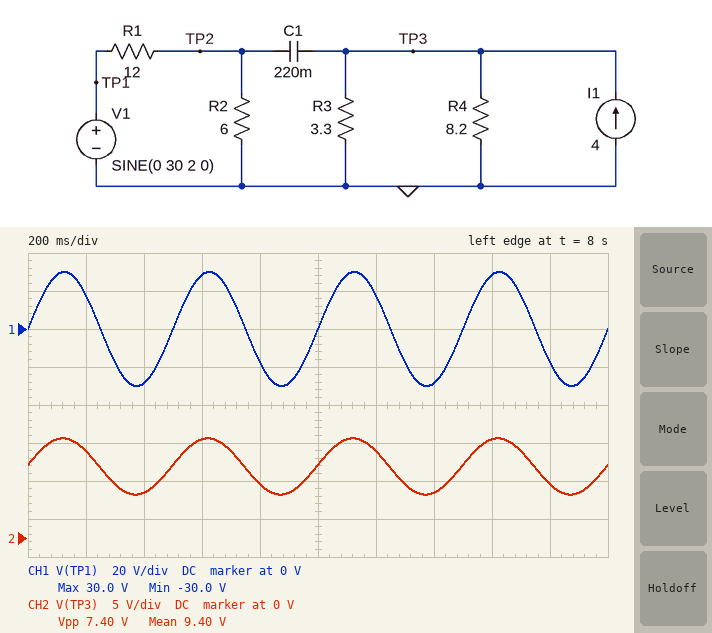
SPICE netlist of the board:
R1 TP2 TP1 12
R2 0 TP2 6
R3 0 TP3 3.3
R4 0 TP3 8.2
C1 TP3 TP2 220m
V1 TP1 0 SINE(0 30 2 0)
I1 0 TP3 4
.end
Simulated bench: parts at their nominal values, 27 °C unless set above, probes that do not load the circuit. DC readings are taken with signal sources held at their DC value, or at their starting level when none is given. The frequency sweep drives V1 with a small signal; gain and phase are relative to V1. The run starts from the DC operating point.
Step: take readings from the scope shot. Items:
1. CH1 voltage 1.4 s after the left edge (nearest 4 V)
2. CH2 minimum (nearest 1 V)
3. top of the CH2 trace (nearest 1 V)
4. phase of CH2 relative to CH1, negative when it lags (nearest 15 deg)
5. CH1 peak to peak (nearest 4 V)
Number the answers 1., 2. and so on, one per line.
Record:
1. -28 V
2. 6 V
3. 13 V
4. 0 deg
5. 60 V
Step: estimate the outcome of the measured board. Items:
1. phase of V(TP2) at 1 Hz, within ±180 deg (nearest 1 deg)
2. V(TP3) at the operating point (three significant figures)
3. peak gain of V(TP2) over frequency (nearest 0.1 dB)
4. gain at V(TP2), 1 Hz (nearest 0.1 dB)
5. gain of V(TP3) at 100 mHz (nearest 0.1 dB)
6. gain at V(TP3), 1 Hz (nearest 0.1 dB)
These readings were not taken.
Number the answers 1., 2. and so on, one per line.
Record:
1. -11 deg
2. 9.41 V
3. -9.5 dB
4. -17.8 dB
5. -21.8 dB
6. -18.2 dB
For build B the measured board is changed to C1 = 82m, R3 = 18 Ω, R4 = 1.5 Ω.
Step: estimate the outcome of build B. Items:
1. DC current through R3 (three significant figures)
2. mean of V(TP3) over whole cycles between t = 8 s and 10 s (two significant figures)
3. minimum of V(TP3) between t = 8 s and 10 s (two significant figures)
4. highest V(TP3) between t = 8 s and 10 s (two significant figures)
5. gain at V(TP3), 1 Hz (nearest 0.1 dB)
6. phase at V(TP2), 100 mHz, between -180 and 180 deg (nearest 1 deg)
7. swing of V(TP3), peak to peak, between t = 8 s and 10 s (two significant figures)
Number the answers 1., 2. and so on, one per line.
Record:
1. 308 mA
2. 5.5 V
3. 3.0 V
4. 8.1 V
5. -21.9 dB
6. -11 deg
7. 5.1 V
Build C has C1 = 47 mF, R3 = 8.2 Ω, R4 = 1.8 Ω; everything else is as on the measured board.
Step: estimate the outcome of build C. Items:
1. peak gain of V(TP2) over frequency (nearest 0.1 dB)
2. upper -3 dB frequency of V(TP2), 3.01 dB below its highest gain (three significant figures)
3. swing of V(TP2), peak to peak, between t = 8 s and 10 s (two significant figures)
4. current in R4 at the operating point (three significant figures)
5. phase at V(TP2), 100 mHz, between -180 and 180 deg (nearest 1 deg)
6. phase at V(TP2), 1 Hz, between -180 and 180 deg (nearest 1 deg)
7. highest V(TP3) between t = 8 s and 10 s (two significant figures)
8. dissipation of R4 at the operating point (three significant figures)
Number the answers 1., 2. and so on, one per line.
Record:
1. -9.5 dB
2. 669 mHz
3. 7.8 V
4. 3.28 A
5. -7 deg
6. -35 deg
7. 8.5 V
8. 19.4 W
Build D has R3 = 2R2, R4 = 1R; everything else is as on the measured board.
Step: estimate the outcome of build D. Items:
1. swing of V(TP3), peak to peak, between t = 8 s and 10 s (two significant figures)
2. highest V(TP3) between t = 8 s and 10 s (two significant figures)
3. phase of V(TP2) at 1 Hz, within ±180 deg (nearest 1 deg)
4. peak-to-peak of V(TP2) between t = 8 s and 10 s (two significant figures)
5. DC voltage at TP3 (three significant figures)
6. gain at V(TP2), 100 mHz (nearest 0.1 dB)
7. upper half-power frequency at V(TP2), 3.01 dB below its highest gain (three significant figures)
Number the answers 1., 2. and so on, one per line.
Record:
1. 2.9 V
2. 4.2 V
3. -38 deg
4. 3.3 V
5. 2.75 V
6. -11.0 dB
7. 158 mHz
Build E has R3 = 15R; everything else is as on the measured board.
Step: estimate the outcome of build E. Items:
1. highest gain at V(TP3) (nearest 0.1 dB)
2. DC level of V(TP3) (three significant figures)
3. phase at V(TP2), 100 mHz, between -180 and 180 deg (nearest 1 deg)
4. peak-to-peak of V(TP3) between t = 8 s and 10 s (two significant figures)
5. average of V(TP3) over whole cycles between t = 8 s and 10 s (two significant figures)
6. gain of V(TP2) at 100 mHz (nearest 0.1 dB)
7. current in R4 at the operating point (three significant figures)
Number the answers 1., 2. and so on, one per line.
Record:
1. -14.4 dB
2. 21.2 V
3. -16 deg
4. 11 V
5. 21 V
6. -11.9 dB
7. 2.59 A
